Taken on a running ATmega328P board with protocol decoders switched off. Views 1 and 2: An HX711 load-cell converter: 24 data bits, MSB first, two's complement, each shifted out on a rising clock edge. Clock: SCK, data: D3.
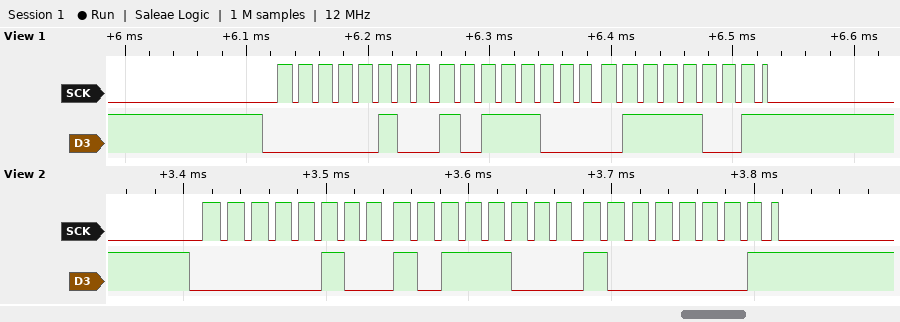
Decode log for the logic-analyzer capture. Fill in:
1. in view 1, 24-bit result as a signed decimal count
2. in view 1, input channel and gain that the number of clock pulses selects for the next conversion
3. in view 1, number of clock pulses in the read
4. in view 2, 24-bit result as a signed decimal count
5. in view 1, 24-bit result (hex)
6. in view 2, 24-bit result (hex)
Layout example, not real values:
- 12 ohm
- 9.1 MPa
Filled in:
- 309369
- channel A, gain 128
- 25
- 309377
- 0x04B879
- 0x04B881
